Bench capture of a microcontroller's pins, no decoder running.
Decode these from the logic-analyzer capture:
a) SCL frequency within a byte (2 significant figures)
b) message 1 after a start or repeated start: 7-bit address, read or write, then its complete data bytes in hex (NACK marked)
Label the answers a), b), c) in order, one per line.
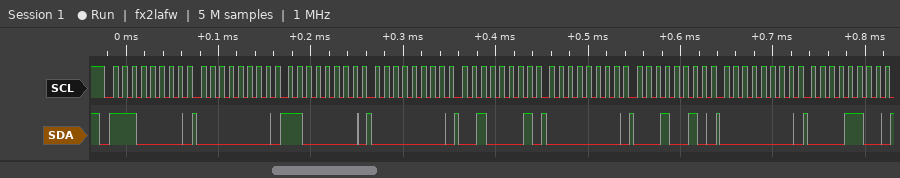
a) 100 kHz
b) 0x70 write: 00 C0 00 21 00 12 00 0C
